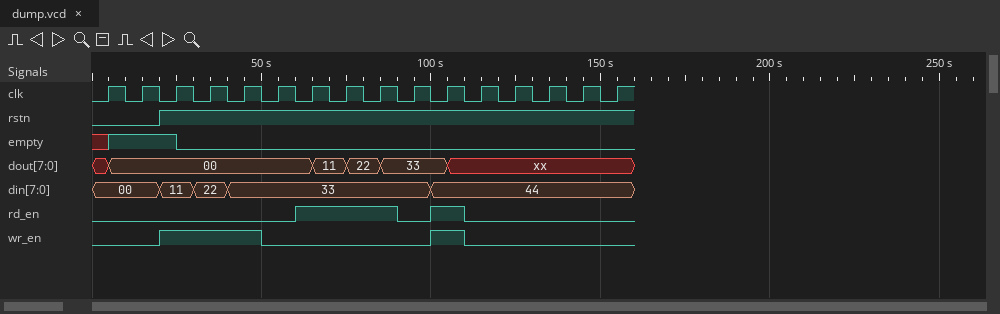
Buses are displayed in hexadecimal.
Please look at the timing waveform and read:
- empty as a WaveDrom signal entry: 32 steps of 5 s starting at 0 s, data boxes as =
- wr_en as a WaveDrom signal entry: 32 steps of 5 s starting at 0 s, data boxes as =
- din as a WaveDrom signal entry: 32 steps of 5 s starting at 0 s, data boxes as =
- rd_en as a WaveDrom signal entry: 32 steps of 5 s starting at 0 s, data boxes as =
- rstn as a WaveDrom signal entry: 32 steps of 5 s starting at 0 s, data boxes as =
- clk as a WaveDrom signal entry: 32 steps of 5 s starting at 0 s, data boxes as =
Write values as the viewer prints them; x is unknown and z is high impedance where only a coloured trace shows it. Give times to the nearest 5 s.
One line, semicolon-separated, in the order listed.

{name: 'empty', wave: 'x1...0..........................'}; {name: 'wr_en', wave: '0...1.....0.........1.0.........'}; {name: 'din', wave: '=...=.=.=...........=...........', data: '00 11 22 33 44'}; {name: 'rd_en', wave: '0...........1.....0.1.0.........'}; {name: 'rstn', wave: '0...1...........................'}; {name: 'clk', wave: '01010101010101010101010101010101'}
